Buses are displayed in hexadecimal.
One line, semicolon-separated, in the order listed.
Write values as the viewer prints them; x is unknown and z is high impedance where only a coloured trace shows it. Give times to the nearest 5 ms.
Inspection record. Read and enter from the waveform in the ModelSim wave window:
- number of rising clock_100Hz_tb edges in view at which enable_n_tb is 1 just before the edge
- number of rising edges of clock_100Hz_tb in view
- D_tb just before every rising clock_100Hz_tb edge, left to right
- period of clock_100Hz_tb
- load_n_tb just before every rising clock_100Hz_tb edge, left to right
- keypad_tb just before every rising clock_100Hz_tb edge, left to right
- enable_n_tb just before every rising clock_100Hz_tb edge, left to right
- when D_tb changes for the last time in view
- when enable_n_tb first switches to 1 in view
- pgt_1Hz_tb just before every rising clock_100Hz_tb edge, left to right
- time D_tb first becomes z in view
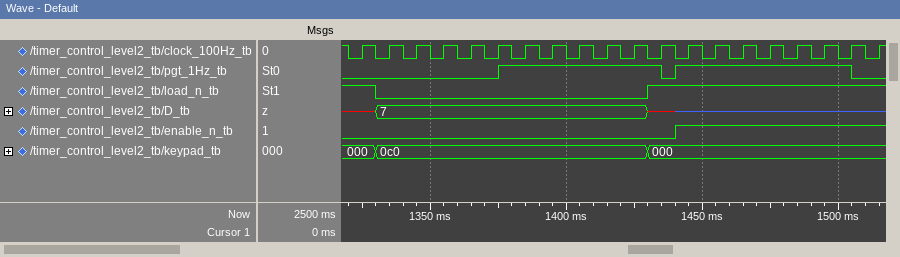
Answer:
8; 20; x, 7, 7, 7, 7, 7, 7, 7, 7, 7, 7, x, z, z, z, z, z, z, z, z; 10 ms; 1 0 0 0 0 0 0 0 0 0 0 1 1 1 1 1 1 1 1 1; 000, 0c0, 0c0, 0c0, 0c0, 0c0, 0c0, 0c0, 0c0, 0c0, 0c0, 000, 000, 000, 000, 000, 000, 000, 000, 000; 0 0 0 0 0 0 0 0 0 0 0 0 1 1 1 1 1 1 1 1; 1440 ms; 1440 ms; 0 0 0 0 0 0 1 1 1 1 1 1 1 1 1 1 1 1 1 0; 1440 ms
